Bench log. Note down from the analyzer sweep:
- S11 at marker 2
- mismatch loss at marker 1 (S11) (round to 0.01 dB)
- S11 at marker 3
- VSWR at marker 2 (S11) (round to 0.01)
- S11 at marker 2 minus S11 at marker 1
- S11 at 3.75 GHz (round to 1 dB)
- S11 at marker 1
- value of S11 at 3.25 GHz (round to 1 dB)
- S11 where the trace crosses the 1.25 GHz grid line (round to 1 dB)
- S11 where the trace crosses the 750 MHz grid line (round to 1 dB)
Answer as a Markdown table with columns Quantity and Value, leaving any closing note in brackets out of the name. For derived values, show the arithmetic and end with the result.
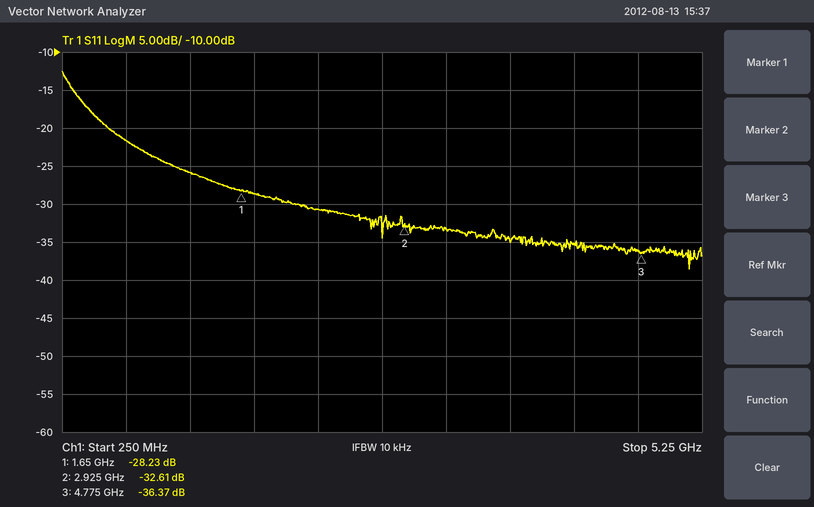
| Quantity | Value |
|---|---|
| S11 at marker 2 | -32.61 dB |
| mismatch loss at marker 1 (S11) | −10 log10(1 − 10^(-28.23/10)) ≈ 0.01 dB |
| S11 at marker 3 | -36.37 dB |
| VSWR at marker 2 (S11) | (1 + 0.0234)/(1 − 0.0234) ≈ 1.05 |
| S11 at marker 2 minus S11 at marker 1 | -32.61 − (-28.23) = -4.38 dB |
| S11 at 3.75 GHz | -35 dB |
| S11 at marker 1 | -28.23 dB |
| value of S11 at 3.25 GHz | -33 dB |
| S11 where the trace crosses the 1.25 GHz grid line | -26 dB |
| S11 where the trace crosses the 750 MHz grid line | -22 dB |
